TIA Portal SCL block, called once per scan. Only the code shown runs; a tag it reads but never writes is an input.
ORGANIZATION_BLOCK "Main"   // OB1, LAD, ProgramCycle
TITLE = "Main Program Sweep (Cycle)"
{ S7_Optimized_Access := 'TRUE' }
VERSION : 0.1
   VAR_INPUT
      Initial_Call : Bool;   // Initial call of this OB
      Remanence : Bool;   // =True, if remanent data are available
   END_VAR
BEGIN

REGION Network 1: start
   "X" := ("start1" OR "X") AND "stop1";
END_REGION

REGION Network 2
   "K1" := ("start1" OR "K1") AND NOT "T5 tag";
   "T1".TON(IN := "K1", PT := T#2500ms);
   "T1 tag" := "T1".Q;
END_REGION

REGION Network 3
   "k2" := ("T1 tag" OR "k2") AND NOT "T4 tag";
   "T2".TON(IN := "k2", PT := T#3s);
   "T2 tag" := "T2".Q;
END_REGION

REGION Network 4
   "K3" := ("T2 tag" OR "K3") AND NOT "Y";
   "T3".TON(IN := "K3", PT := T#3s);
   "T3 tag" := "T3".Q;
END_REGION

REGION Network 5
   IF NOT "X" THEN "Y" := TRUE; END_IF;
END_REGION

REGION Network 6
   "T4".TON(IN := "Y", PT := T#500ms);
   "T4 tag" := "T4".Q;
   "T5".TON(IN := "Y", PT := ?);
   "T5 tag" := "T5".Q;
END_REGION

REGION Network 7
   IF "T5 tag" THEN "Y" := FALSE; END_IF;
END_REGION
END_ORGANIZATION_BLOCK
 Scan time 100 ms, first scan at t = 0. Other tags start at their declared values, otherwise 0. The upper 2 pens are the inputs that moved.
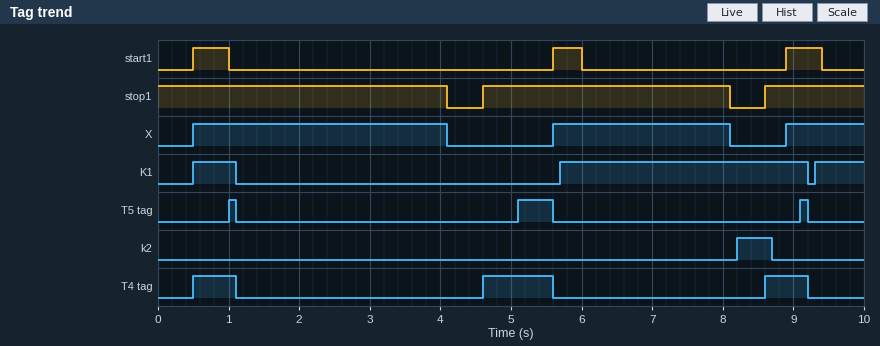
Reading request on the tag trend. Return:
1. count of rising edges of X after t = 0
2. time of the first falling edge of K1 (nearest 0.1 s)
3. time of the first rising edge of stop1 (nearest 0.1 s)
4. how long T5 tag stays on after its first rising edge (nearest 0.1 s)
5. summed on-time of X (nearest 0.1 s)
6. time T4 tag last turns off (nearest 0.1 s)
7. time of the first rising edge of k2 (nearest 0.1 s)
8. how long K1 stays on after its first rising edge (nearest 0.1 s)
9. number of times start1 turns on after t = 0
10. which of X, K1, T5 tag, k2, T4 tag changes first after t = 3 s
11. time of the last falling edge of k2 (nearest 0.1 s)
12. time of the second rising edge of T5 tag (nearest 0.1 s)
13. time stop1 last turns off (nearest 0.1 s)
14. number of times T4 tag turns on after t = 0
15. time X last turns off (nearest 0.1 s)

3
1.1 s
4.6 s
0.1 s
7.2 s
9.2 s
8.2 s
0.6 s
3
X
8.7 s
5.1 s
8.1 s
3
8.1 s
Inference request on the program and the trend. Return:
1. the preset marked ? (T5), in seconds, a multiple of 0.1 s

1.0 s
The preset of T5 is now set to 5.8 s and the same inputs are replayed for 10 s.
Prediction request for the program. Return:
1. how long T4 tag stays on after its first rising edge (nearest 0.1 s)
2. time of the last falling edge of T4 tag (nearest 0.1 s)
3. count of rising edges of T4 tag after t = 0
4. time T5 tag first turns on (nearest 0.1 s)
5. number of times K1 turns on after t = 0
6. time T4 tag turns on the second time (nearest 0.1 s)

5.4 s
5.9 s
2
5.8 s
2
8.6 s
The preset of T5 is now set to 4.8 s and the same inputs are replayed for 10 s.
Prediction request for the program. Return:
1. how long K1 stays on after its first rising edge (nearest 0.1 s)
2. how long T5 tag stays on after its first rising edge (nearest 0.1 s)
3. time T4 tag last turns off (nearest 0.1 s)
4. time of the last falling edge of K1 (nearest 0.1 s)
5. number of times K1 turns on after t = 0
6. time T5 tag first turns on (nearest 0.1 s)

4.4 s
0.8 s
5.6 s
4.9 s
2
4.8 s
